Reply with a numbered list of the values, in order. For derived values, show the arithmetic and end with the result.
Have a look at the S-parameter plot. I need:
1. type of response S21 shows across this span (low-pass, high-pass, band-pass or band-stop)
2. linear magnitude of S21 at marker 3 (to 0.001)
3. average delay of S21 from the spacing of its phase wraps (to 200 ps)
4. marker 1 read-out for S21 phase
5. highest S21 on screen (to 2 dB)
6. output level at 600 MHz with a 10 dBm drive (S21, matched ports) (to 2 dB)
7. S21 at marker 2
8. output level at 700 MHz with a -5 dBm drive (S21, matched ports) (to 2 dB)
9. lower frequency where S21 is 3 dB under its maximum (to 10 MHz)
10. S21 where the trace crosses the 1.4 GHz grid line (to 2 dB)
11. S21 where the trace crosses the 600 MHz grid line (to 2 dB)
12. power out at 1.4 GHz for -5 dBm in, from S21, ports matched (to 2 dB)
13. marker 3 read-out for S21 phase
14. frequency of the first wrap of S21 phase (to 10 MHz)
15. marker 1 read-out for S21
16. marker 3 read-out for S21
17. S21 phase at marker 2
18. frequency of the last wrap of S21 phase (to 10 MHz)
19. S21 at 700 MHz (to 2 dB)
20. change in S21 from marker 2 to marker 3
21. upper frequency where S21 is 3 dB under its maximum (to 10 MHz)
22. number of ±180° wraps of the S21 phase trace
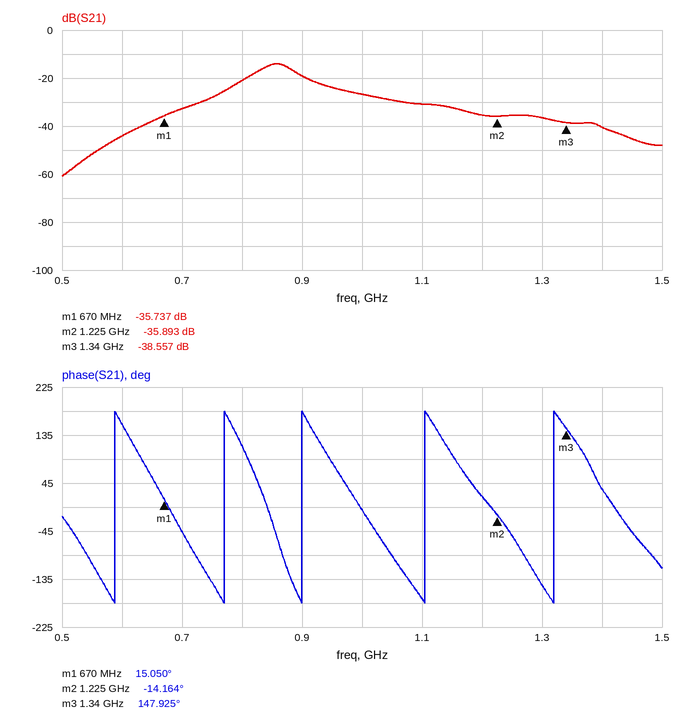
1. band-pass
2. 10^(-38.557/20) ≈ 0.012
3. 4 cycles / (1.32 GHz − 590 MHz) ≈ 5.48 ns, so 5.4 ns to the nearest 200 ps
4. 15.050°
5. -14 dB
6. 10 dBm + (-44 dB) = -34 dBm
7. -35.893 dB
8. -5 dBm + (-32 dB) = -38 dBm
9. 830 MHz
10. -40 dB
11. -44 dB
12. -5 dBm + (-40 dB) = -46 dBm
13. 147.925°
14. 590 MHz
15. -35.737 dB
16. -38.557 dB
17. -14.164°
18. 1.32 GHz
19. -32 dB
20. -38.557 − (-35.893) = -2.664 dB
21. 890 MHz
22. 5
